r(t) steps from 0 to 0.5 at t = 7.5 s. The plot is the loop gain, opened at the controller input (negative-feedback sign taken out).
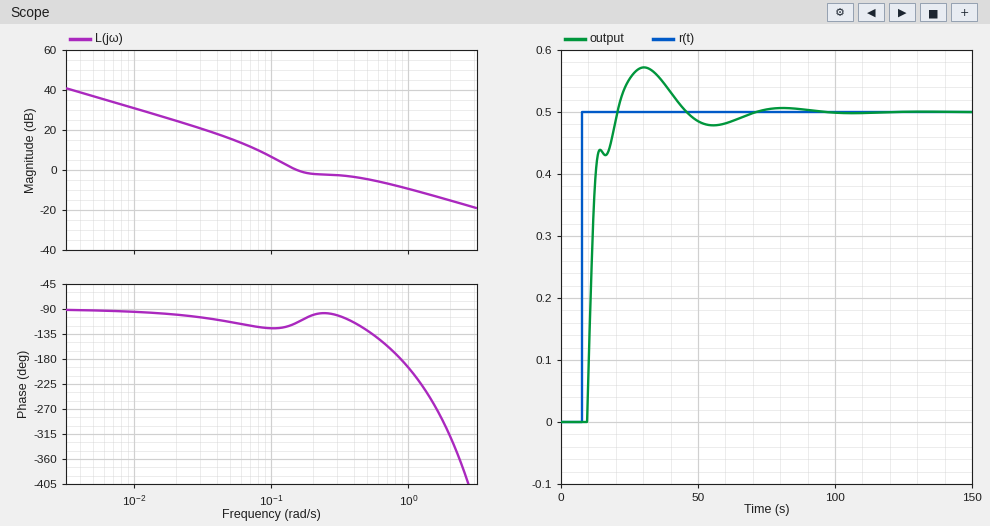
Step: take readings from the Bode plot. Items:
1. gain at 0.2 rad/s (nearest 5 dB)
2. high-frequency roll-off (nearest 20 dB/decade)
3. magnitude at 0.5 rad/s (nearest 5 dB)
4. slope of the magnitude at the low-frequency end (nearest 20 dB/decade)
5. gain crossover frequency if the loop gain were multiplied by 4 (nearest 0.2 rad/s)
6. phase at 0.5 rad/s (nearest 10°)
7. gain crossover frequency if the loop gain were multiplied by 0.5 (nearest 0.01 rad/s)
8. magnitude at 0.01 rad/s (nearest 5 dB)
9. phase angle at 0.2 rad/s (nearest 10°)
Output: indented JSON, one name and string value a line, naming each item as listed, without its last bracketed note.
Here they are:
{
  "gain at 0.2 rad/s": "0 dB",
  "high-frequency roll-off": "-20 dB/decade",
  "magnitude at 0.5 rad/s": "-5 dB",
  "slope of the magnitude at the low-frequency end": "-20 dB/decade",
  "gain crossover frequency if the loop gain were multiplied by 4": "1.4 rad/s",
  "phase at 0.5 rad/s": "-130°",
  "gain crossover frequency if the loop gain were multiplied by 0.5": "0.10 rad/s",
  "magnitude at 0.01 rad/s": "30 dB",
  "phase angle at 0.2 rad/s": "-100°"
}
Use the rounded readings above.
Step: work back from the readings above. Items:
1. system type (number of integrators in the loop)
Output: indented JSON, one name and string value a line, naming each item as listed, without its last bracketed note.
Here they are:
{
  "system type": "1"
}
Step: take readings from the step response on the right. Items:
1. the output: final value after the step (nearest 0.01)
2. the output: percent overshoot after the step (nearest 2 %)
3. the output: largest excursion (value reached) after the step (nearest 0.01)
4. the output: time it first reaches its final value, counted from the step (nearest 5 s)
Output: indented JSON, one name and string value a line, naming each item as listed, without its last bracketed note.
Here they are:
{
  "the output: final value after the step": "0.50",
  "the output: percent overshoot after the step": "14 %",
  "the output: largest excursion (value reached) after the step": "0.57",
  "the output: time it first reaches its final value, counted from the step": "15 s"
}
